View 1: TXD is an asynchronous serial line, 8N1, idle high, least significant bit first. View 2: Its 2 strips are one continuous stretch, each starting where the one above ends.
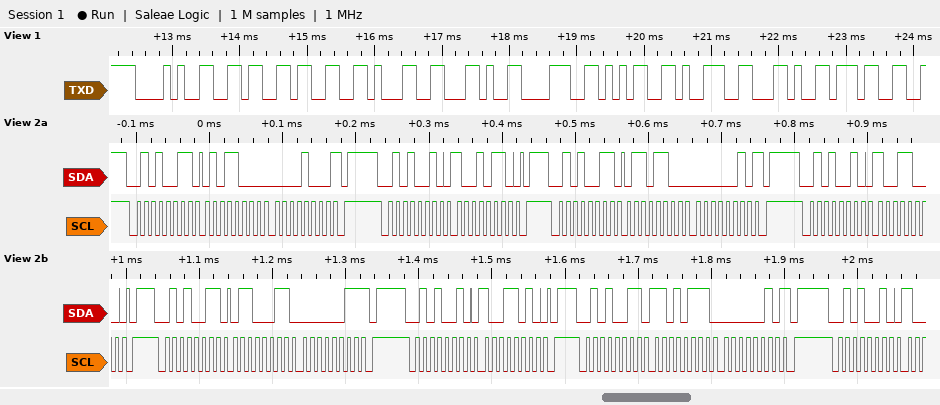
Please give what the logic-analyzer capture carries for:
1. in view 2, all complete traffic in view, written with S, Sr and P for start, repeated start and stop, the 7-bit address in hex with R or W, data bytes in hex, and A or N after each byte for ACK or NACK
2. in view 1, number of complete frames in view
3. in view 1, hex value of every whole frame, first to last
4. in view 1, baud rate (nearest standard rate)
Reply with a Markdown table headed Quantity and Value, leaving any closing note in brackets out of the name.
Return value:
| Quantity | Value |
|---|---|
| in view 2, all complete traffic in view, written with S, Sr and P for start, repeated start and stop, the 7-bit address in hex with R or W, data bytes in hex, and A or N after each byte for ACK or NACK | S 29R A 58 A 08 N P S 29W A 96 A P S 29R A 6C A 02 N P S 29W A 98 A P S 29R A 63 A 03 N P S 29W A 9A A P S 29R A D7 A 02 N P S 29W A |
| in view 1, number of complete frames in view | 10 |
| in view 1, hex value of every whole frame, first to last | 28 36 33 31 2C 38 35 39 2C 37 |
| in view 1, baud rate | 9600 baud |
